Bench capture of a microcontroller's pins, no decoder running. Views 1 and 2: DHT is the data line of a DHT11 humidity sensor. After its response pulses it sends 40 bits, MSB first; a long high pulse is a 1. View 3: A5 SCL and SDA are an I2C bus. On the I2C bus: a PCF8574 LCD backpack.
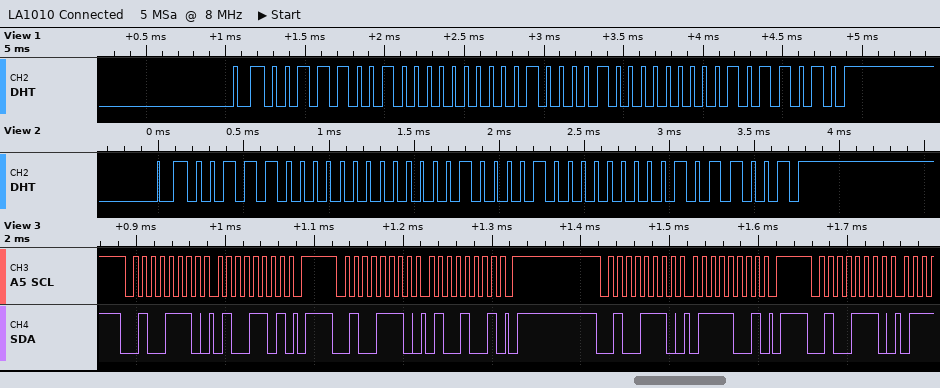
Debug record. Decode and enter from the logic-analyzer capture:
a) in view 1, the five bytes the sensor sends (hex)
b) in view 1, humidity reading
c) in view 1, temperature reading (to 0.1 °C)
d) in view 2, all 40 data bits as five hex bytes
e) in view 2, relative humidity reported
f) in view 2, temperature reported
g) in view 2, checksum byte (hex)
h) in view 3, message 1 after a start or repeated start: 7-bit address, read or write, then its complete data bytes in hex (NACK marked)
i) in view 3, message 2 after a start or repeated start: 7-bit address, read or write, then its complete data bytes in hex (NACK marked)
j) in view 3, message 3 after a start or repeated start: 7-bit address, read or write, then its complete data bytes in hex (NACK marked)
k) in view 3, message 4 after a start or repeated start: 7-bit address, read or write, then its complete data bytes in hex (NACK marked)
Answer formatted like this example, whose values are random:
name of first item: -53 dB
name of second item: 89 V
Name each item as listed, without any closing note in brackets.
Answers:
in view 1, the five bytes the sensor sends: 39 00 21 00 5A
in view 1, humidity reading: 57 %
in view 1, temperature reading: 33.0 °C
in view 2, all 40 data bits as five hex bytes: 38 00 21 00 59
in view 2, relative humidity reported: 56 %
in view 2, temperature reported: 33.0 °C
in view 2, checksum byte: 0x59
in view 3, message 1 after a start or repeated start: 7-bit address, read or write, then its complete data bytes in hex: 0x27 write: 4D
in view 3, message 2 after a start or repeated start: 7-bit address, read or write, then its complete data bytes in hex: 0x27 write: 49
in view 3, message 3 after a start or repeated start: 7-bit address, read or write, then its complete data bytes in hex: 0x27 write: 79
in view 3, message 4 after a start or repeated start: 7-bit address, read or write, then its complete data bytes in hex: 0x27 write
